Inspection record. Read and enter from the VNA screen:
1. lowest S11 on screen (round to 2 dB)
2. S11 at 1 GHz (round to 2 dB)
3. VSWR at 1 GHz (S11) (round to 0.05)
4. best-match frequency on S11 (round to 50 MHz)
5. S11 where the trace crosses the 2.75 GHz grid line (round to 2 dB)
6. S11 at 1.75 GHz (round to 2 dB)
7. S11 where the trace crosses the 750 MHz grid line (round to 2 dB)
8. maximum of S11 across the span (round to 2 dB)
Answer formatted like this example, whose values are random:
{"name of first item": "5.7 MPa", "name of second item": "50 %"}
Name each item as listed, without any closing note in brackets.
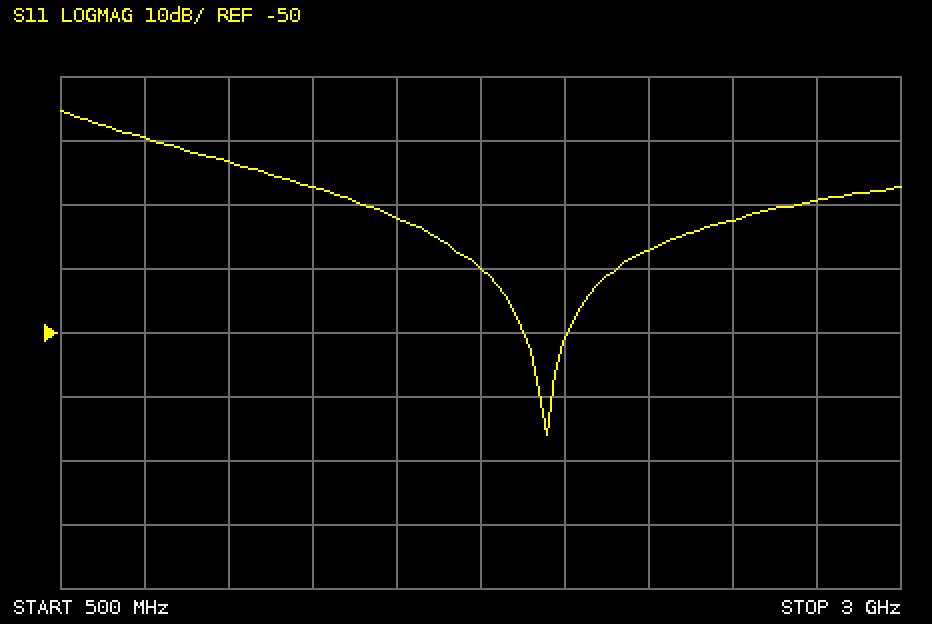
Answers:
{"lowest S11 on screen": "-66 dB", "S11 at 1 GHz": "-24 dB", "VSWR at 1 GHz (S11)": "1.15", "best-match frequency on S11": "1.95 GHz", "S11 where the trace crosses the 2.75 GHz grid line": "-30 dB", "S11 at 1.75 GHz": "-40 dB", "S11 where the trace crosses the 750 MHz grid line": "-20 dB", "maximum of S11 across the span": "-16 dB"}
